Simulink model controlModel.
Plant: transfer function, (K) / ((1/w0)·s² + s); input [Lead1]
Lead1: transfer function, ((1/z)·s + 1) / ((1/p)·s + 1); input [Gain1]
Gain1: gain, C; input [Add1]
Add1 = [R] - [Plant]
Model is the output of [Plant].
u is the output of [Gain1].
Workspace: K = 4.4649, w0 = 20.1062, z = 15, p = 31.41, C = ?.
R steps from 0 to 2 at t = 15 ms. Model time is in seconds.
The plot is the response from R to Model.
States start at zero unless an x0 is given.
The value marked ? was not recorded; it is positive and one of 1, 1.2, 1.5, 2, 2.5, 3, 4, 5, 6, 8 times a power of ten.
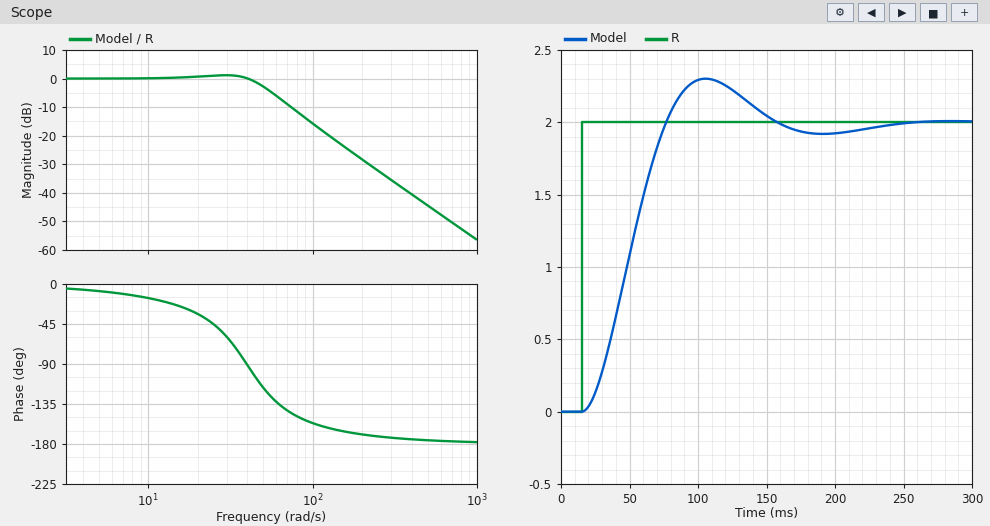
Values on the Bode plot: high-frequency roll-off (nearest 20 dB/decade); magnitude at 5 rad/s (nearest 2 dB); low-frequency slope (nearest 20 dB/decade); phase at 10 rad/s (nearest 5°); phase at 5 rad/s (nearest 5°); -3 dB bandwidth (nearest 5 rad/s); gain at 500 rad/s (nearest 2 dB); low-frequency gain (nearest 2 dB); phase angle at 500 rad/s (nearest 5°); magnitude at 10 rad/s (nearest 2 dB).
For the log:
-40 dB/decade
0 dB
0 dB/decade
-15°
-10°
50 rad/s
-44 dB
0 dB
-175°
0 dB
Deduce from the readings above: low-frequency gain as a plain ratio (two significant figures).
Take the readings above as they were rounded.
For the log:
1.0
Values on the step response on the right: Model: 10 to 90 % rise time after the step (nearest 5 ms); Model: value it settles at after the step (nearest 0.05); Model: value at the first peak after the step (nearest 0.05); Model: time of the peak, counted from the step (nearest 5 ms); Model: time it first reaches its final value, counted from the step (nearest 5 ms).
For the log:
40 ms
2.00
2.30
90 ms
60 ms
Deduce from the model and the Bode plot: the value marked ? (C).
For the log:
8
